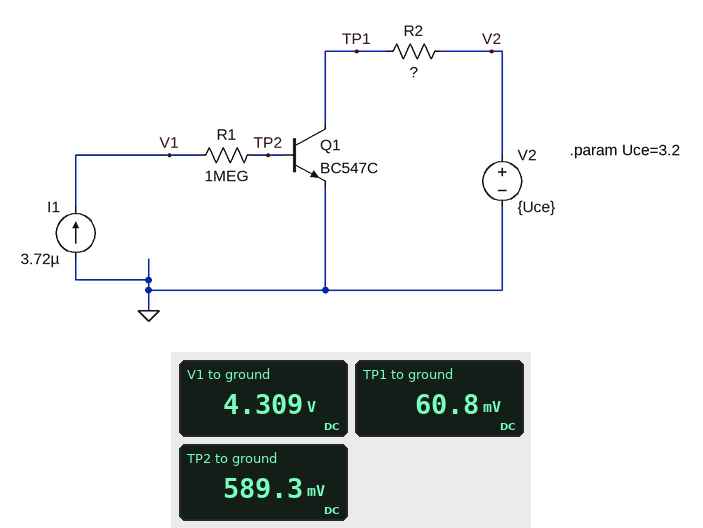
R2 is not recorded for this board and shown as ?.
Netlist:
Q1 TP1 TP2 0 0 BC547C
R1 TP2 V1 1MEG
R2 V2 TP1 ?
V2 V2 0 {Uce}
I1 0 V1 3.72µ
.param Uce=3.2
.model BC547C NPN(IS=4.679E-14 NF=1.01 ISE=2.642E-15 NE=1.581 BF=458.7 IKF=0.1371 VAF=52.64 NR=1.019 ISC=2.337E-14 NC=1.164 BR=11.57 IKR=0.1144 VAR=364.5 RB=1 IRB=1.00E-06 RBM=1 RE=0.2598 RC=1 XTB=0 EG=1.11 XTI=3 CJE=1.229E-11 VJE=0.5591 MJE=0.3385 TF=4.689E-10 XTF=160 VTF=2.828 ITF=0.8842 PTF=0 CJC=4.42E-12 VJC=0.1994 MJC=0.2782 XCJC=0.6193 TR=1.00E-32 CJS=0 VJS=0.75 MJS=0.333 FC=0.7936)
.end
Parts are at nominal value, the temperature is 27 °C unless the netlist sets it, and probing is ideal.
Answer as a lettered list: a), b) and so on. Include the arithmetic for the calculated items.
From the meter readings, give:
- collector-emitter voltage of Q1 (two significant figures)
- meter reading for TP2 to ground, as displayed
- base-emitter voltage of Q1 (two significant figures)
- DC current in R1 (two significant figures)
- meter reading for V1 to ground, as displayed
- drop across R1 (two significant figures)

a) 60.8 mV = 61 mV
b) 589.3 mV
c) 589.3 mV = 590 mV
d) (4.309 V - 589.3 mV) / 1 MΩ = 3.7 µA
e) 4.309 V
f) 4.309 V - 589.3 mV = 3.7 V
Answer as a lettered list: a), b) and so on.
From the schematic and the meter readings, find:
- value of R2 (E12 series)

a) 12 kΩ
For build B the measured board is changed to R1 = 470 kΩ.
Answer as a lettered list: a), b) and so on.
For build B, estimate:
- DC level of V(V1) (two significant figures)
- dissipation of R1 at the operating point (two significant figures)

a) 2.3 V
b) 6.5 µW
